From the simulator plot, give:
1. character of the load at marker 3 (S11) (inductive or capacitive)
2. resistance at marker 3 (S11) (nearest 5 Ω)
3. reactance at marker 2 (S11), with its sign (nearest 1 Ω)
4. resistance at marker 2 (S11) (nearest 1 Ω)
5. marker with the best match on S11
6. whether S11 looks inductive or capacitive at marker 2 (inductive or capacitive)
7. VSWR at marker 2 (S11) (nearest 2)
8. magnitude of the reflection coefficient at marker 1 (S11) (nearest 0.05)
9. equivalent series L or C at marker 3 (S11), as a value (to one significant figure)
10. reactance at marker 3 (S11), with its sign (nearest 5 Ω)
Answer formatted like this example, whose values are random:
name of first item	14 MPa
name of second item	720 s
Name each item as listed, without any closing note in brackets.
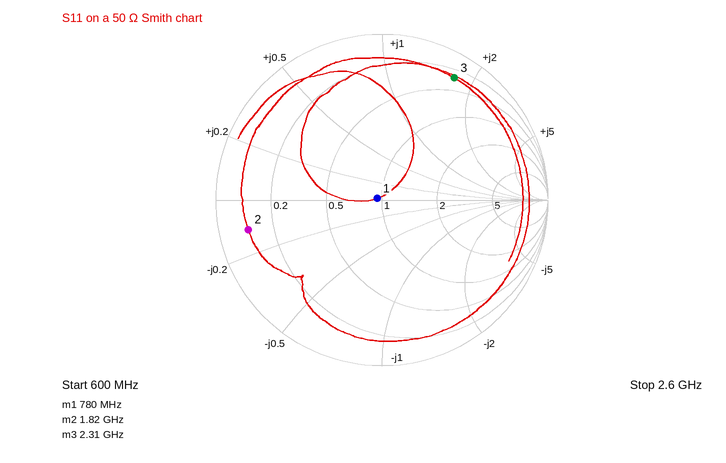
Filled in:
character of the load at marker 3 (S11)	inductive
resistance at marker 3 (S11)	15 Ω
reactance at marker 2 (S11), with its sign	-5 Ω
resistance at marker 2 (S11)	5 Ω
marker with the best match on S11	marker 1
whether S11 looks inductive or capacitive at marker 2	capacitive
VSWR at marker 2 (S11)	10
magnitude of the reflection coefficient at marker 1 (S11)	0.05
equivalent series L or C at marker 3 (S11), as a value	6 nH
reactance at marker 3 (S11), with its sign	+85 Ω
